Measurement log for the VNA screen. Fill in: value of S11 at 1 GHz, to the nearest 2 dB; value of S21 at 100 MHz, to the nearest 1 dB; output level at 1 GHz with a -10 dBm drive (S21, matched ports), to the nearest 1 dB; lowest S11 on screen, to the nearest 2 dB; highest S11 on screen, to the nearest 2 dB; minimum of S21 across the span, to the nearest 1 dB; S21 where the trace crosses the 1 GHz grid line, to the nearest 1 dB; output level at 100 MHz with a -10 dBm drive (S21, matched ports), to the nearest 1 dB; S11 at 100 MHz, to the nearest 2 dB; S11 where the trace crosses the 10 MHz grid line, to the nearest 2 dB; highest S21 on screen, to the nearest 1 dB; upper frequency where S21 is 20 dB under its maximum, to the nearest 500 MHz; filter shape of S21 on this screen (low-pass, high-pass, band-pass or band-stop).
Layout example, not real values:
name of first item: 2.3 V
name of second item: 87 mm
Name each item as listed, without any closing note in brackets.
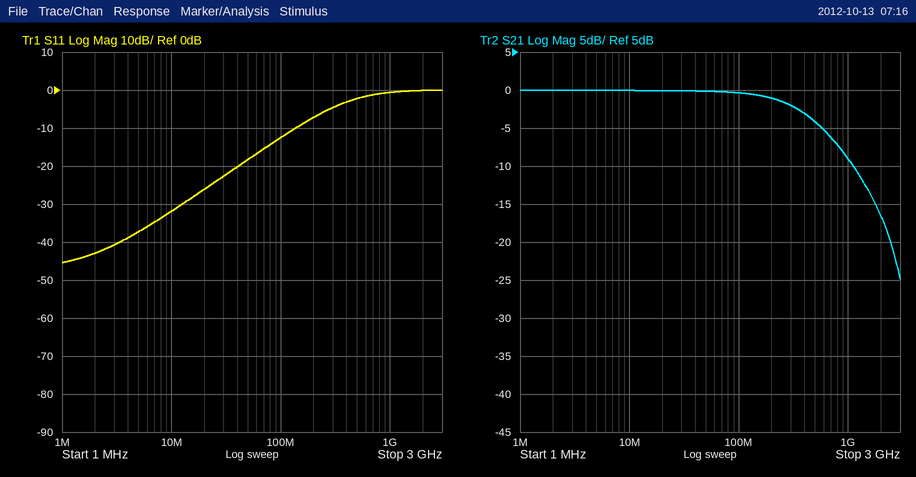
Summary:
value of S11 at 1 GHz, to the nearest 2 dB: 0 dB
value of S21 at 100 MHz, to the nearest 1 dB: 0 dB
output level at 1 GHz with a -10 dBm drive (S21, matched ports), to the nearest 1 dB: -19 dBm
lowest S11 on screen, to the nearest 2 dB: -46 dB
highest S11 on screen, to the nearest 2 dB: 0 dB
minimum of S21 across the span, to the nearest 1 dB: -25 dB
S21 where the trace crosses the 1 GHz grid line, to the nearest 1 dB: -9 dB
output level at 100 MHz with a -10 dBm drive (S21, matched ports), to the nearest 1 dB: -10 dBm
S11 at 100 MHz, to the nearest 2 dB: -12 dB
S11 where the trace crosses the 10 MHz grid line, to the nearest 2 dB: -32 dB
highest S21 on screen, to the nearest 1 dB: 0 dB
upper frequency where S21 is 20 dB under its maximum, to the nearest 500 MHz: 2.5 GHz
filter shape of S21 on this screen: low-pass
